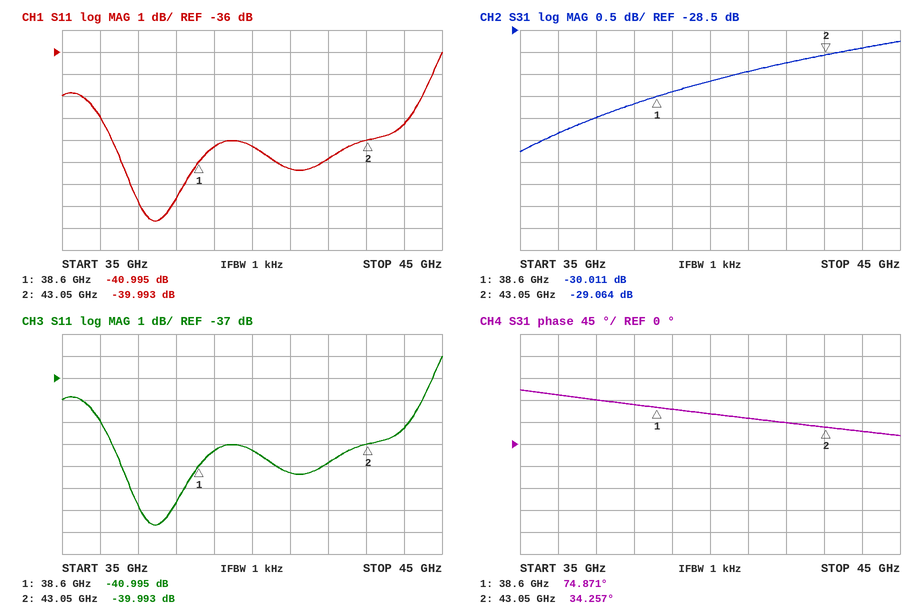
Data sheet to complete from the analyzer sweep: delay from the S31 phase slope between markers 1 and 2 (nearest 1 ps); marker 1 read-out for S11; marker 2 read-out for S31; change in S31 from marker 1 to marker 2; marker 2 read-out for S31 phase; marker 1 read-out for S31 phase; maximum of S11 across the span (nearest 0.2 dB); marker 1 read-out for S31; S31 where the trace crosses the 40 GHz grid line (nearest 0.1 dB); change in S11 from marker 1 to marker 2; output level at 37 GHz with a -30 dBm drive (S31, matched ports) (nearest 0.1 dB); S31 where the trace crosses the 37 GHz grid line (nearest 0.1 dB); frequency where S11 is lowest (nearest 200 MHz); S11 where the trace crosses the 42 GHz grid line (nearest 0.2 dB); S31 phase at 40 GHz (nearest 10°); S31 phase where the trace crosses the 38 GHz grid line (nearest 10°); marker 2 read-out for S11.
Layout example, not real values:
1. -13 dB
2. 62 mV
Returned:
1. 25 ps
2. -40.995 dB
3. -29.064 dB
4. 0.947 dB
5. 34.257°
6. 74.871°
7. -36.0 dB
8. -30.011 dB
9. -29.7 dB
10. 1.002 dB
11. -60.5 dBm
12. -30.5 dB
13. 37.4 GHz
14. -40.8 dB
15. 60°
16. 80°
17. -39.993 dB
